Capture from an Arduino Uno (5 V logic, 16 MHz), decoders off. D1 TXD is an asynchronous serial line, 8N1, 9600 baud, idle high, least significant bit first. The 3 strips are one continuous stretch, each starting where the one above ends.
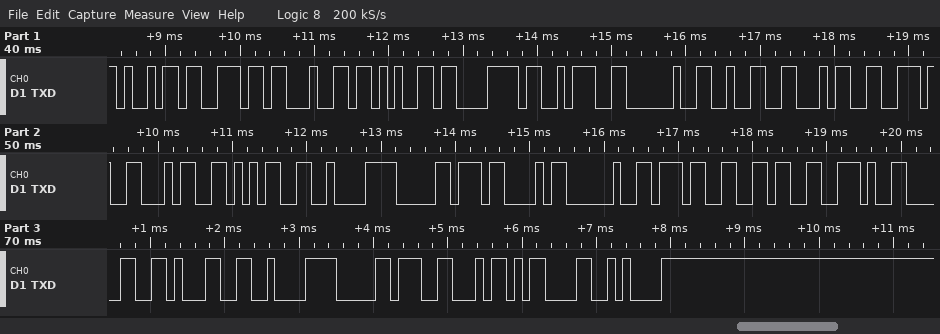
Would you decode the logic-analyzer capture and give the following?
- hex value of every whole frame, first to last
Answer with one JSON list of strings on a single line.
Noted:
["69 6E 64 65 78 3A 20 32 34 2E 34 35 C2 B0 43 20 37 36 2E 30 31 C2 B0 46 0D 0A"]
